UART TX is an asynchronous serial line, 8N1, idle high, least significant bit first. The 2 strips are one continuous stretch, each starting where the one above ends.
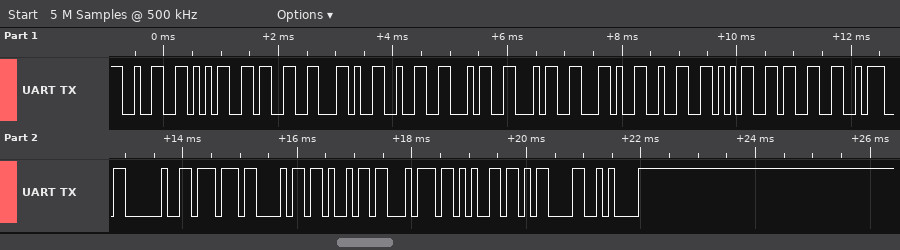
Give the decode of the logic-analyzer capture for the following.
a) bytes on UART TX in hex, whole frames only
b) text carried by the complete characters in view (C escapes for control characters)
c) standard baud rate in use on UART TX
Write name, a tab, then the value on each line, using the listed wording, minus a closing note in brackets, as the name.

bytes on UART TX in hex, whole frames only	32 35 33 2C 32 34 34 2C 32 35 33 3A 20 77 68 69 74 65 0D 0A
text carried by the complete characters in view	"253,244,253: white\r\n"
standard baud rate in use on UART TX	9600 baud
